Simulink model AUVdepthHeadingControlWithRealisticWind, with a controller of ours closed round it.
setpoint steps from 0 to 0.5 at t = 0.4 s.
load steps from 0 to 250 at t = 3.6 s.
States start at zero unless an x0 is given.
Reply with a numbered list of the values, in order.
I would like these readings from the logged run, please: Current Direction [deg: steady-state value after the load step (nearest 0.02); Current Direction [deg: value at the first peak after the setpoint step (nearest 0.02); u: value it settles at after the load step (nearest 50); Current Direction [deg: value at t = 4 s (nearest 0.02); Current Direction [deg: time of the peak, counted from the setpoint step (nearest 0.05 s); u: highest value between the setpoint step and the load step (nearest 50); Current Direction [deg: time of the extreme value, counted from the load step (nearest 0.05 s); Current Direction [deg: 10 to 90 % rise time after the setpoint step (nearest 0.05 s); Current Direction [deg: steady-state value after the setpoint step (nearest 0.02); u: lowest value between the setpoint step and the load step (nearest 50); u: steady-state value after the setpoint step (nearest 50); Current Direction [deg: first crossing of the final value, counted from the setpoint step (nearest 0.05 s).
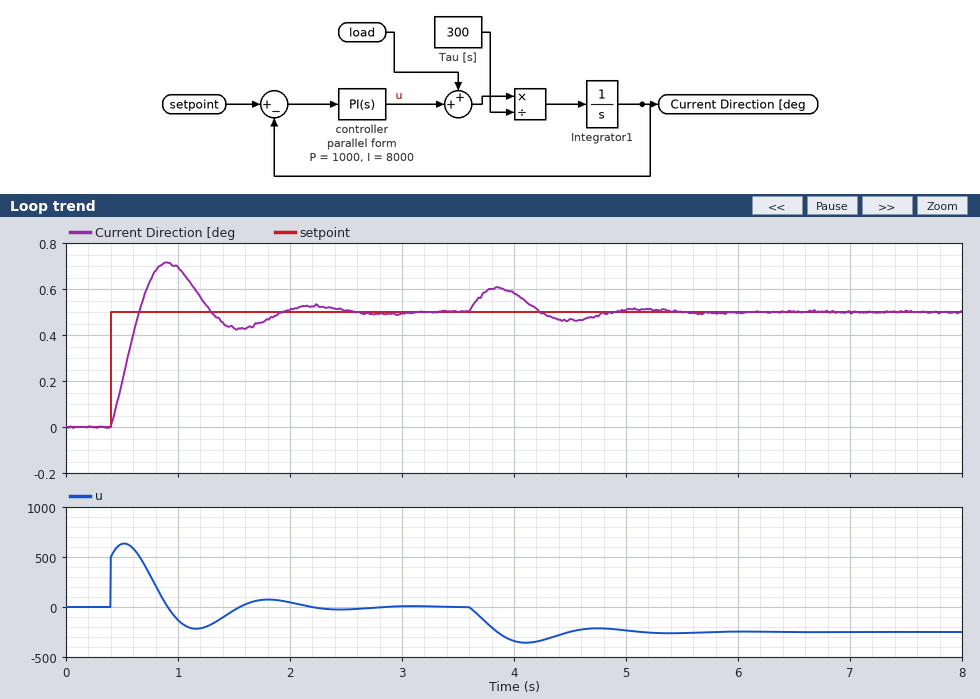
1. 0.50
2. 0.72
3. -250
4. 0.58
5. 0.50 s
6. 650
7. 0.25 s
8. 0.20 s
9. 0.50
10. -200
11. 0
12. 0.25 s
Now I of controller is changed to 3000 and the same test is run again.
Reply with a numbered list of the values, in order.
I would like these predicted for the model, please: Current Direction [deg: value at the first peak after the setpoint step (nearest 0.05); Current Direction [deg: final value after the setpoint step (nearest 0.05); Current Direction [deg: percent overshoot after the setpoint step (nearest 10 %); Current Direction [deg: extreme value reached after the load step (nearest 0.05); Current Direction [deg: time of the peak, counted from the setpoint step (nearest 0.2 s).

1. 0.65
2. 0.50
3. 30 %
4. 0.65
5. 0.8 s
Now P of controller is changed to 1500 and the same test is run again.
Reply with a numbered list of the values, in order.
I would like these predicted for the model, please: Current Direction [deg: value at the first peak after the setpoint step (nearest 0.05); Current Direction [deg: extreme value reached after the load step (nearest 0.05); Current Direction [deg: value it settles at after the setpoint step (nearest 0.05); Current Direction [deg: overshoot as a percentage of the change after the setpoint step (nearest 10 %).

1. 0.65
2. 0.60
3. 0.50
4. 30 %
